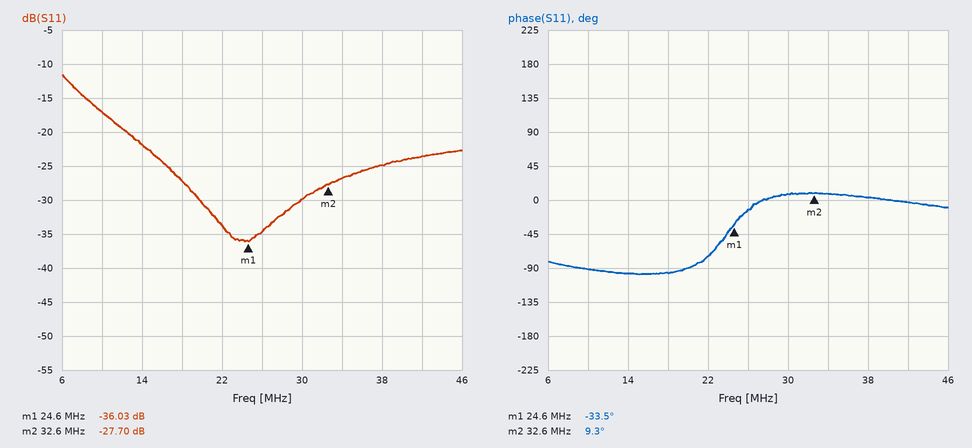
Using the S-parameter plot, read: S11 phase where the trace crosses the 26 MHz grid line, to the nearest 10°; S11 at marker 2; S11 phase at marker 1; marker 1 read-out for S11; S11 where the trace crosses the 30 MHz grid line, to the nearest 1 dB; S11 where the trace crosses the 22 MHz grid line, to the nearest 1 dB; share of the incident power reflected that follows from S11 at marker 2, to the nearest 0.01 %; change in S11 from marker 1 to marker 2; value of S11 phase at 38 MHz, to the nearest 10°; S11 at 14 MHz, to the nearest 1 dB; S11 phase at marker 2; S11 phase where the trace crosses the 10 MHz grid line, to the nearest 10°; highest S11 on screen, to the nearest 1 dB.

-10°
-27.70 dB
-33.5°
-36.03 dB
-30 dB
-34 dB
0.17 %
8.33 dB
0°
-22 dB
9.3°
-90°
-12 dB
